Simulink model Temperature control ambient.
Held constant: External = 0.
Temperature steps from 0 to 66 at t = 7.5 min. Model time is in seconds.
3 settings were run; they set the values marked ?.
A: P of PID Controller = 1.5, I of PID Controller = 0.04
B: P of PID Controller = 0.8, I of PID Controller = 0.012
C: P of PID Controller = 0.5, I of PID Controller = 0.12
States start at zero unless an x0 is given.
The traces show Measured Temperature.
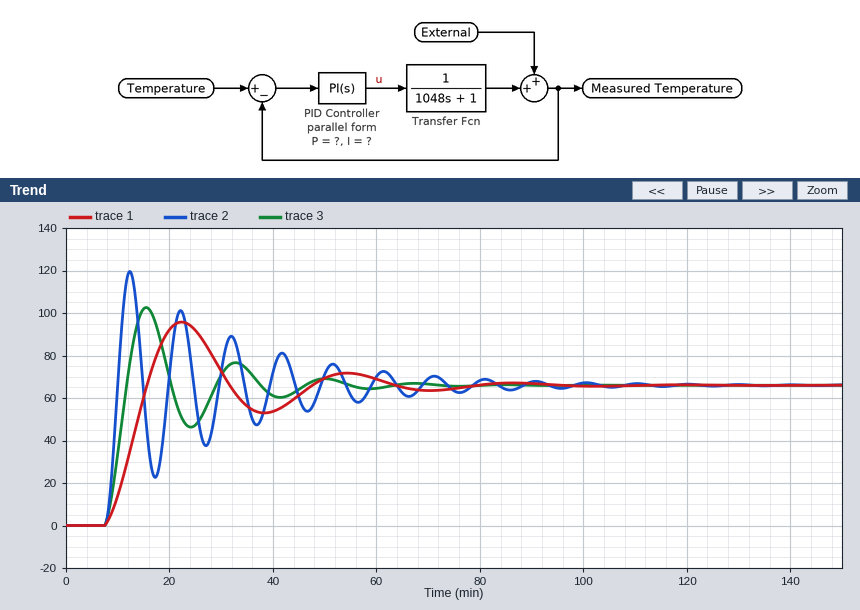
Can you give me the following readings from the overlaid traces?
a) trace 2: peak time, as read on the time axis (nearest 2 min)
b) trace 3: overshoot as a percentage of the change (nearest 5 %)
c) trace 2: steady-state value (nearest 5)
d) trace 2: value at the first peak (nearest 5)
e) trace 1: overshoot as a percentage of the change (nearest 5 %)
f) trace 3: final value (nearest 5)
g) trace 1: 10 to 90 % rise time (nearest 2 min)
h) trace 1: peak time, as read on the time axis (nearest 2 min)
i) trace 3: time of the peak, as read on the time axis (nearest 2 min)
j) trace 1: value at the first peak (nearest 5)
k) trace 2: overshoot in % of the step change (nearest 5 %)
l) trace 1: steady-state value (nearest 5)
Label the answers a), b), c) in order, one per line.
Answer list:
a) 12 min
b) 55 %
c) 65
d) 120
e) 45 %
f) 65
g) 6 min
h) 22 min
i) 16 min
j) 95
k) 80 %
l) 65
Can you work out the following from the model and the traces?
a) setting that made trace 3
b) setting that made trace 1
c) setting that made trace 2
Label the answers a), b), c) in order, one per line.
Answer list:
a) A
b) B
c) C
